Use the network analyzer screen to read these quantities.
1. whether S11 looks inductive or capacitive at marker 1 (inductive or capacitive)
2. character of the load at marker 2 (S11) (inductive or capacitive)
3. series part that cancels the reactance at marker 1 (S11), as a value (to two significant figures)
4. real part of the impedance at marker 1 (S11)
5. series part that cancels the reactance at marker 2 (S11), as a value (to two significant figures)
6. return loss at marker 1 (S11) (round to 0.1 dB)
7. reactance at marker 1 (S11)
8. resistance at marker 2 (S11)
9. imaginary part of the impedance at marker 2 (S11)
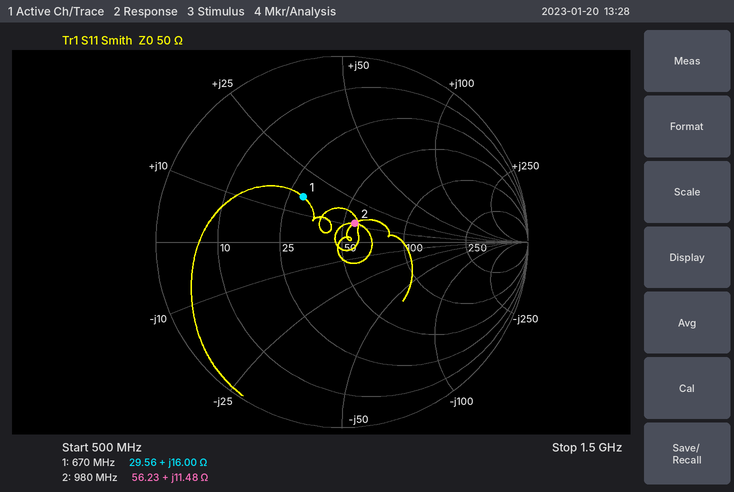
inductive
inductive
15 pF
29.56 Ω
14 pF
9.9 dB
+16.00 Ω
56.23 Ω
+11.48 Ω
